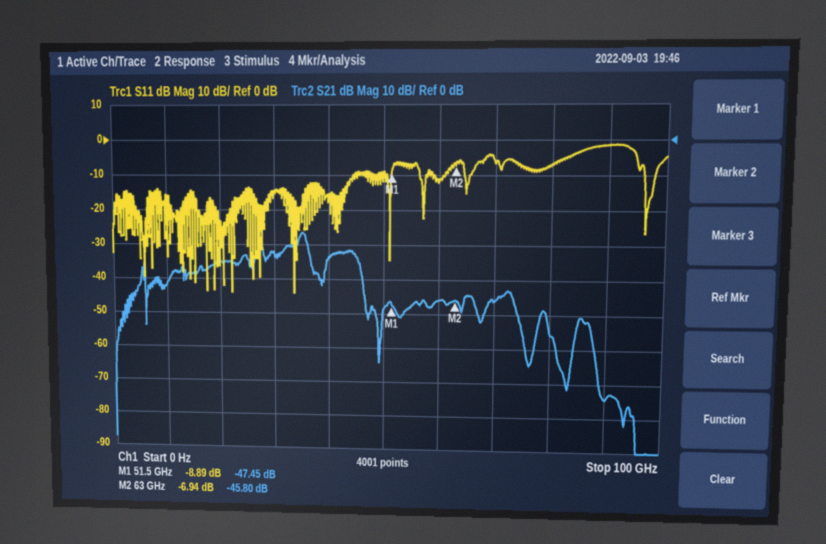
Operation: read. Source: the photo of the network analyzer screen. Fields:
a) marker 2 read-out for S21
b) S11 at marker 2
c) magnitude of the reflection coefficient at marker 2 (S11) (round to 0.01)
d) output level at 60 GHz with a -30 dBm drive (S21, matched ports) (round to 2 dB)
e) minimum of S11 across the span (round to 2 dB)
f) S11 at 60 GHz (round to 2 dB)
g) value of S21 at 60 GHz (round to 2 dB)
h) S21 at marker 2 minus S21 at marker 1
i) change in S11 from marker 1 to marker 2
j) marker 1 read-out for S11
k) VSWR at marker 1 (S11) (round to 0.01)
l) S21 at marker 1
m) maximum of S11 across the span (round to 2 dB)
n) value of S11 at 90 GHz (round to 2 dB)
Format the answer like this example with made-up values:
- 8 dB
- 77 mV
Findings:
- -45.80 dB
- -6.94 dB
- 0.45
- -76 dBm
- -44 dB
- -12 dB
- -46 dB
- 1.65 dB
- 1.95 dB
- -8.89 dB
- 2.12
- -47.45 dB
- -2 dB
- -2 dB
